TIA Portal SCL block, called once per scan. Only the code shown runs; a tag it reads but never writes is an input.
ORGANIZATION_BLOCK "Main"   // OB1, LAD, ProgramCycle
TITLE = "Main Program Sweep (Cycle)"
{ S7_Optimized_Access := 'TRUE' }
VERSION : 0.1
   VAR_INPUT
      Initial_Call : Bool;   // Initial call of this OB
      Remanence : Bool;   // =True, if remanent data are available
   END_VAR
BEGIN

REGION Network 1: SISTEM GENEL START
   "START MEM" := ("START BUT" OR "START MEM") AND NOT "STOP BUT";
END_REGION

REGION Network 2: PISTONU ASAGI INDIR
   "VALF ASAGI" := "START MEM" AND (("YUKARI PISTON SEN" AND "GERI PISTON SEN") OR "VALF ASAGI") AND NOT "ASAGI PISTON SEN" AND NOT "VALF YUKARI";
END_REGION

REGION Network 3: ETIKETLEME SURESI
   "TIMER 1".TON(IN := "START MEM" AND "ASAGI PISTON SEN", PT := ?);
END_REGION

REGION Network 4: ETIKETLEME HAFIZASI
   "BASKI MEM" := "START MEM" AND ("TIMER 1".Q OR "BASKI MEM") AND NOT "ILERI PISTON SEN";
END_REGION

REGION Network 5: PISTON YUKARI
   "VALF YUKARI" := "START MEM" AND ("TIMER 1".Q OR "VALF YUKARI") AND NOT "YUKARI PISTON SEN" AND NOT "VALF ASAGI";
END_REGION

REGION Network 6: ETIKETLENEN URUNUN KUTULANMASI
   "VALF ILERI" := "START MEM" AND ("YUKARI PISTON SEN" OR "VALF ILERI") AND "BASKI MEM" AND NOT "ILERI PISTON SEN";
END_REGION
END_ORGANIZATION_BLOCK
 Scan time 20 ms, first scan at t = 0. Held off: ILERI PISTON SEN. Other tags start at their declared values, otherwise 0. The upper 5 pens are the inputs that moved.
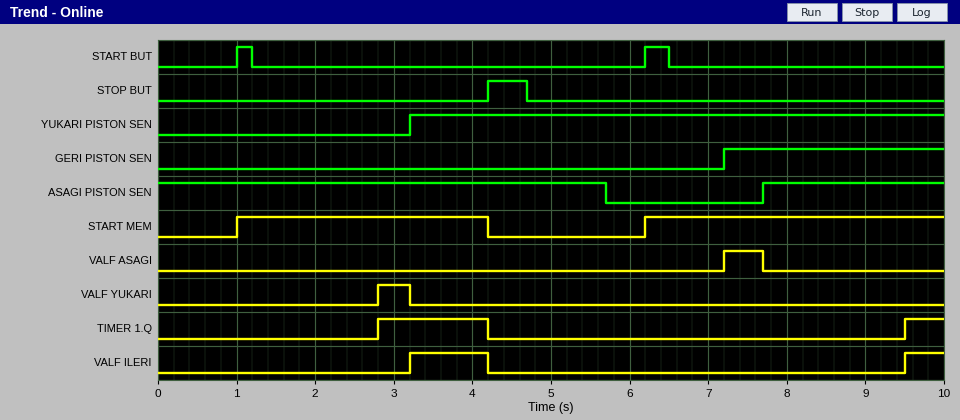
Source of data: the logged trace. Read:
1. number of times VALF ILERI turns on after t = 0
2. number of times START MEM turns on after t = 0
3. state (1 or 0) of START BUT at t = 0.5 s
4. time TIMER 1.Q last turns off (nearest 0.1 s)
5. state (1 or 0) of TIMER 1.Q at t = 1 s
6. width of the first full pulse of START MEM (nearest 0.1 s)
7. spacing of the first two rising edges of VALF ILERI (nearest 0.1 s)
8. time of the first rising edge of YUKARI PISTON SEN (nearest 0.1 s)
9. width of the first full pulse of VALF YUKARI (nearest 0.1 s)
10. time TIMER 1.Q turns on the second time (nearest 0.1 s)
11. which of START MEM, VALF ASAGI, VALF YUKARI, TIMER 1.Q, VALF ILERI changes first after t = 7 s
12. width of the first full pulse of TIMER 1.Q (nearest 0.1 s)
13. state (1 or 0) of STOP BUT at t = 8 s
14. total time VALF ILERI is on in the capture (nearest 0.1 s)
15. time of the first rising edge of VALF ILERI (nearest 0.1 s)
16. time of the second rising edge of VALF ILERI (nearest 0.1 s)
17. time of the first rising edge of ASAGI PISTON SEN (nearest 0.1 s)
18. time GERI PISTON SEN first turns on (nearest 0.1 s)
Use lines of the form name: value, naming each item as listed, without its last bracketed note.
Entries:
number of times VALF ILERI turns on after t = 0: 2
number of times START MEM turns on after t = 0: 2
state (1 or 0) of START BUT at t = 0.5 s: 0
time TIMER 1.Q last turns off: 4.2 s
state (1 or 0) of TIMER 1.Q at t = 1 s: 0
width of the first full pulse of START MEM: 3.2 s
spacing of the first two rising edges of VALF ILERI: 6.3 s
time of the first rising edge of YUKARI PISTON SEN: 3.2 s
width of the first full pulse of VALF YUKARI: 0.4 s
time TIMER 1.Q turns on the second time: 9.5 s
which of START MEM, VALF ASAGI, VALF YUKARI, TIMER 1.Q, VALF ILERI changes first after t = 7 s: VALF ASAGI
width of the first full pulse of TIMER 1.Q: 1.4 s
state (1 or 0) of STOP BUT at t = 8 s: 0
total time VALF ILERI is on in the capture: 1.5 s
time of the first rising edge of VALF ILERI: 3.2 s
time of the second rising edge of VALF ILERI: 9.5 s
time of the first rising edge of ASAGI PISTON SEN: 7.7 s
time GERI PISTON SEN first turns on: 7.2 s
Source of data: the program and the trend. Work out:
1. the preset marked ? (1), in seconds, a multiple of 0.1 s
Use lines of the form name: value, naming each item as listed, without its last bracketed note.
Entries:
the preset marked ? (1), in seconds, a multiple of 0.1 s: 1.8 s
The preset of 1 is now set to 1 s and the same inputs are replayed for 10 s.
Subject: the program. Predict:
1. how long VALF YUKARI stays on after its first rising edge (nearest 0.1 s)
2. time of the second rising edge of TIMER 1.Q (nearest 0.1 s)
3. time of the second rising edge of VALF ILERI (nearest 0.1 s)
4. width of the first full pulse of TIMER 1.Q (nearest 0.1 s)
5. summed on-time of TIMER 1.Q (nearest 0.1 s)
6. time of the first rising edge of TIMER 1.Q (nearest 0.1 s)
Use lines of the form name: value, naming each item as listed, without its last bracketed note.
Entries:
how long VALF YUKARI stays on after its first rising edge: 1.2 s
time of the second rising edge of TIMER 1.Q: 8.7 s
time of the second rising edge of VALF ILERI: 8.7 s
width of the first full pulse of TIMER 1.Q: 2.2 s
summed on-time of TIMER 1.Q: 3.5 s
time of the first rising edge of TIMER 1.Q: 2.0 s
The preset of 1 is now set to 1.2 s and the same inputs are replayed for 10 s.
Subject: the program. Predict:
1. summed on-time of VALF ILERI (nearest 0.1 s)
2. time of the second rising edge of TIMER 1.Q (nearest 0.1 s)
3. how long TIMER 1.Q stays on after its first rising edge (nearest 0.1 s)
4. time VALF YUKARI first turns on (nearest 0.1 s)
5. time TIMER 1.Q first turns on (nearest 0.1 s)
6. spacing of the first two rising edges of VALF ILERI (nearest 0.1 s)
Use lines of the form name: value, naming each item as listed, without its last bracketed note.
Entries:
summed on-time of VALF ILERI: 2.1 s
time of the second rising edge of TIMER 1.Q: 8.9 s
how long TIMER 1.Q stays on after its first rising edge: 2.0 s
time VALF YUKARI first turns on: 2.2 s
time TIMER 1.Q first turns on: 2.2 s
spacing of the first two rising edges of VALF ILERI: 5.7 s
